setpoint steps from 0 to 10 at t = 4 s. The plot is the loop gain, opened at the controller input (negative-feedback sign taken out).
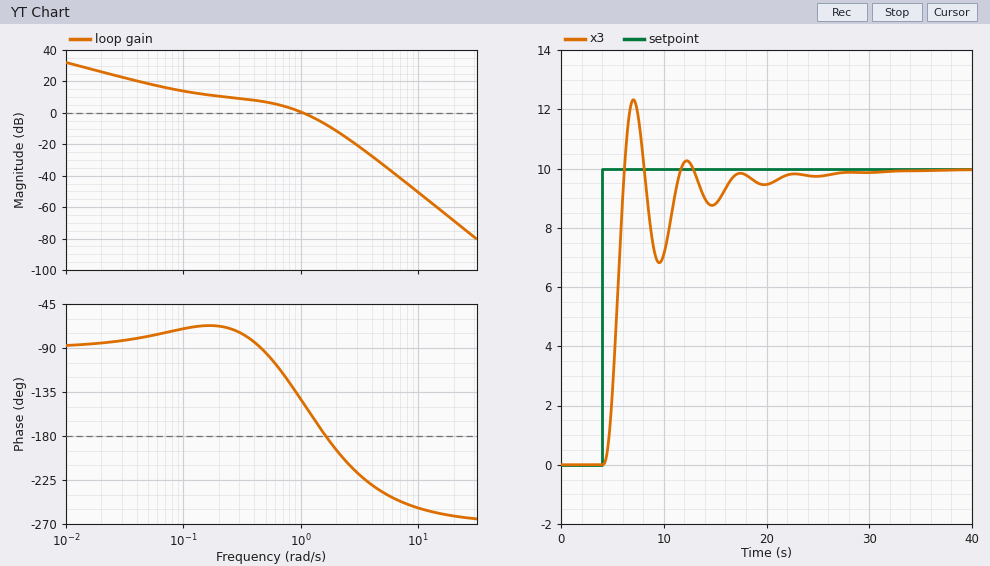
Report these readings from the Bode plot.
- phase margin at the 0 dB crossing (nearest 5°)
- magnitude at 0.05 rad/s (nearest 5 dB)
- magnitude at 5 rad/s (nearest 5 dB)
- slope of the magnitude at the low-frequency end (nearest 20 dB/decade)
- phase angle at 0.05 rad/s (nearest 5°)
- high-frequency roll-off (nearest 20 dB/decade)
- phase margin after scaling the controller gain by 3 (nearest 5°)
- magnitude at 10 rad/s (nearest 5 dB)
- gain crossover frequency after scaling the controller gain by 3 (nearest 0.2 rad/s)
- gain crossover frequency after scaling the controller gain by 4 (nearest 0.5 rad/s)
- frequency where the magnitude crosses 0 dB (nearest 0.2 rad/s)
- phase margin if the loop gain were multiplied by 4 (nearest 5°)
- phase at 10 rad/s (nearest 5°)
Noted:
35°
20 dB
-35 dB
-20 dB/decade
-80°
-60 dB/decade
-10°
-50 dB
1.8 rad/s
2.0 rad/s
1.0 rad/s
-15°
-255°
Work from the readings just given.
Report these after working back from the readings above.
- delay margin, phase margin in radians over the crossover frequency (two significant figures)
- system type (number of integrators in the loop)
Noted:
0.61 s
1
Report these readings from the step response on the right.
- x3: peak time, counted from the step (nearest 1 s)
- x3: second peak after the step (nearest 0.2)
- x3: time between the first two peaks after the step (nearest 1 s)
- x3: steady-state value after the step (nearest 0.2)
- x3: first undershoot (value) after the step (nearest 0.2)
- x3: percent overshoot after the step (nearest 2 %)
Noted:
3 s
10.2
5 s
10.0
6.8
24 %
